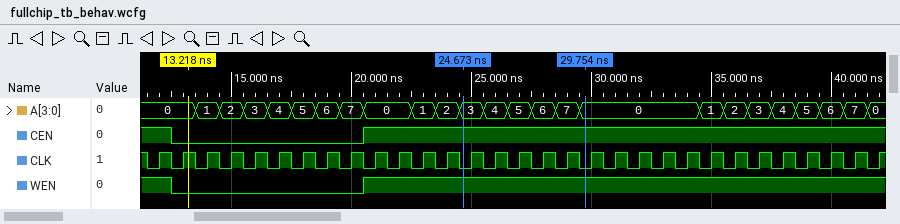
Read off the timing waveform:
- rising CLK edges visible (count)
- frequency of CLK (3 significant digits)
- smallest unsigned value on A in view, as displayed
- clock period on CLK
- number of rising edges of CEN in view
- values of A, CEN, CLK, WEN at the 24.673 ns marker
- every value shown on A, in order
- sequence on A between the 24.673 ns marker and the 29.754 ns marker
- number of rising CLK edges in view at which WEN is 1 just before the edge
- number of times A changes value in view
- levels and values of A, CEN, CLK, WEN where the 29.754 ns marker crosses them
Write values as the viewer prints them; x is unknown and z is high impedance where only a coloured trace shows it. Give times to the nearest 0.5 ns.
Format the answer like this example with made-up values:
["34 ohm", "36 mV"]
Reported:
["31", "1.00 GHz", "0", "1 ns", "1", "A=3, CEN=1, CLK=0, WEN=1", "0, 1, 2, 3, 4, 5, 6, 7, 0, 1, 2, 3, 4, 5, 6, 7, 0, 1, 2, 3, 4, 5, 6, 7, 0", "3, 4, 5, 6, 7, 0", "23", "24", "A=0, CEN=1, CLK=0, WEN=1"]
